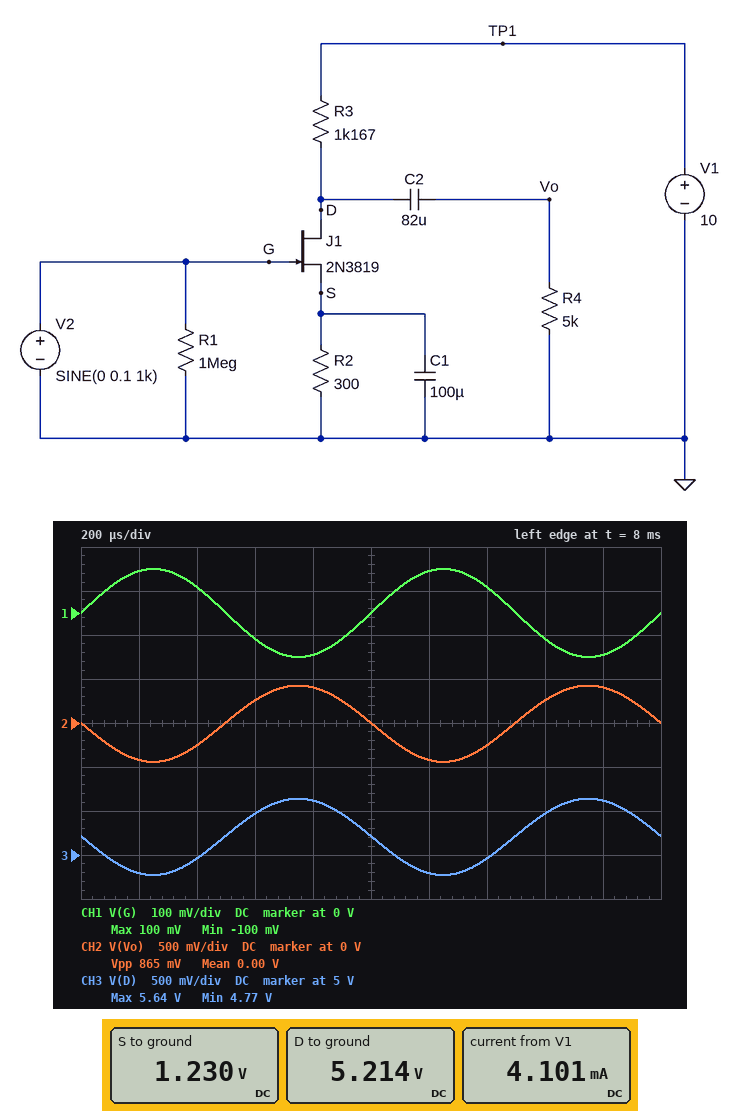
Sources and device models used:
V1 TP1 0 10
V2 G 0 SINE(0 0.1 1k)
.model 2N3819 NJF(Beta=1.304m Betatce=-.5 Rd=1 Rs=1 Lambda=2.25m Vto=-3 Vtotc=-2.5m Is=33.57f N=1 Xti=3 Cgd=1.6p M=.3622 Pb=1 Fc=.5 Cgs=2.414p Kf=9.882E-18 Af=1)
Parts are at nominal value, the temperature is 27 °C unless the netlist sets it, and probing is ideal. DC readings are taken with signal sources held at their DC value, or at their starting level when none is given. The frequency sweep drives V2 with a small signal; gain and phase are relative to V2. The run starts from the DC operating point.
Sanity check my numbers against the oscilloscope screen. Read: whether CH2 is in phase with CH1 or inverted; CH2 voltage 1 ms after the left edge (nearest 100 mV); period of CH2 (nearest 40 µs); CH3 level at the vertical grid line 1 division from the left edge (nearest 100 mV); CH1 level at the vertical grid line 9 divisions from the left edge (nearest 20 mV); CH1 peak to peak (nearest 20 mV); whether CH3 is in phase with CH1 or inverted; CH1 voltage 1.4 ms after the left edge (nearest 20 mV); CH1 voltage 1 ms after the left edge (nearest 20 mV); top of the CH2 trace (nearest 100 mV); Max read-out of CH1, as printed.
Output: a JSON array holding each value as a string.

["inverted", "0 V", "1.00 ms", "4.8 V", "-100 mV", "200 mV", "inverted", "60 mV", "0 V", "400 mV", "100 mV"]
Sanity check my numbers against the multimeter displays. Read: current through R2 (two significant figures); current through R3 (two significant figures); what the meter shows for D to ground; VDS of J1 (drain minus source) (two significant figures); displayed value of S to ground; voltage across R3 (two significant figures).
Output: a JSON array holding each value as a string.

["4.1 mA", "4.1 mA", "5.214 V", "4.0 V", "1.230 V", "4.8 V"]
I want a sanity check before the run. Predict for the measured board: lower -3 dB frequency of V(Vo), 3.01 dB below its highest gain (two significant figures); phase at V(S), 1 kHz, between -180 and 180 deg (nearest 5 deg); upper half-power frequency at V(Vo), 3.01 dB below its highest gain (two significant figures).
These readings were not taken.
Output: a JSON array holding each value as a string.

["10 Hz", "-90 deg", "280 MHz"]
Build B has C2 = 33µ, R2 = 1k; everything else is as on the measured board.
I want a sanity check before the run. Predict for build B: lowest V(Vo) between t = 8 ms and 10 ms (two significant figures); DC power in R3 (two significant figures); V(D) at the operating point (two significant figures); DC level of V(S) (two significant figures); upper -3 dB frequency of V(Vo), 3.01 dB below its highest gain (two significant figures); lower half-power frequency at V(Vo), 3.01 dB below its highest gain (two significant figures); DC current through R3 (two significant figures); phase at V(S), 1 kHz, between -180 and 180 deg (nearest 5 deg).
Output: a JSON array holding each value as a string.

["-300 mV", "3.9 mW", "7.9 V", "1.8 V", "360 MHz", "6.2 Hz", "1.8 mA", "-90 deg"]
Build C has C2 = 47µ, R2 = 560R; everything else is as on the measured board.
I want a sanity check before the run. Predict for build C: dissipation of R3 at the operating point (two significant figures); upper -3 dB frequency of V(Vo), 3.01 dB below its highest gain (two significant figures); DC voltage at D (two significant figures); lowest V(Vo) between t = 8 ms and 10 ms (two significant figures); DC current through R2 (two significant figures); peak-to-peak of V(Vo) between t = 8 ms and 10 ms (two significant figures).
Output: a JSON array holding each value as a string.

["8.9 mW", "320 MHz", "6.8 V", "-370 mV", "2.8 mA", "720 mV"]
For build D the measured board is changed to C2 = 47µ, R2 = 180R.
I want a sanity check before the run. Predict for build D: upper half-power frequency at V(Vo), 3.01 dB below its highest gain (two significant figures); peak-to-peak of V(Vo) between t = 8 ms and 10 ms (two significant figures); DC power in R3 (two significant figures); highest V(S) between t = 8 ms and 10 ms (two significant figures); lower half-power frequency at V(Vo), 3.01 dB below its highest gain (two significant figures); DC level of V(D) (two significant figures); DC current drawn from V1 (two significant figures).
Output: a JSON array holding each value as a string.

["240 MHz", "990 mV", "34 mW", "970 mV", "12 Hz", "3.7 V", "5.4 mA"]
